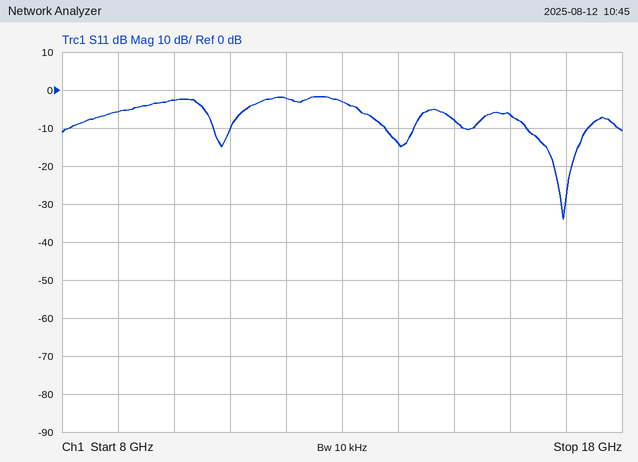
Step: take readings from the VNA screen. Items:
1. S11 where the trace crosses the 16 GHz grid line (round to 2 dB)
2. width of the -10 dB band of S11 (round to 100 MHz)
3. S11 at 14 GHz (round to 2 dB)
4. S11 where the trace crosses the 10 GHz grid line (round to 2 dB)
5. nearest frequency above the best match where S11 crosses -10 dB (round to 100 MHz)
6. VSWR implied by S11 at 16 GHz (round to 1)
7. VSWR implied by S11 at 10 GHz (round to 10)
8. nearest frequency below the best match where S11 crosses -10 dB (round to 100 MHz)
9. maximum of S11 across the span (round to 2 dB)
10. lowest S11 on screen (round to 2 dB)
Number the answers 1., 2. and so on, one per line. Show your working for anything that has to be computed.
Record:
1. -6 dB
2. 17.4 GHz − 16.3 GHz = 1.1 GHz
3. -14 dB
4. -2 dB
5. 17.4 GHz
6. |Γ| = 10^(-6/20) = 0.5012; VSWR = (1 + 0.5012)/(1 − 0.5012) ≈ 3
7. |Γ| = 10^(-2/20) = 0.7943; VSWR = (1 + 0.7943)/(1 − 0.7943) ≈ 8.72, so 10 to the nearest 10
8. 16.3 GHz
9. -2 dB
10. -34 dB
